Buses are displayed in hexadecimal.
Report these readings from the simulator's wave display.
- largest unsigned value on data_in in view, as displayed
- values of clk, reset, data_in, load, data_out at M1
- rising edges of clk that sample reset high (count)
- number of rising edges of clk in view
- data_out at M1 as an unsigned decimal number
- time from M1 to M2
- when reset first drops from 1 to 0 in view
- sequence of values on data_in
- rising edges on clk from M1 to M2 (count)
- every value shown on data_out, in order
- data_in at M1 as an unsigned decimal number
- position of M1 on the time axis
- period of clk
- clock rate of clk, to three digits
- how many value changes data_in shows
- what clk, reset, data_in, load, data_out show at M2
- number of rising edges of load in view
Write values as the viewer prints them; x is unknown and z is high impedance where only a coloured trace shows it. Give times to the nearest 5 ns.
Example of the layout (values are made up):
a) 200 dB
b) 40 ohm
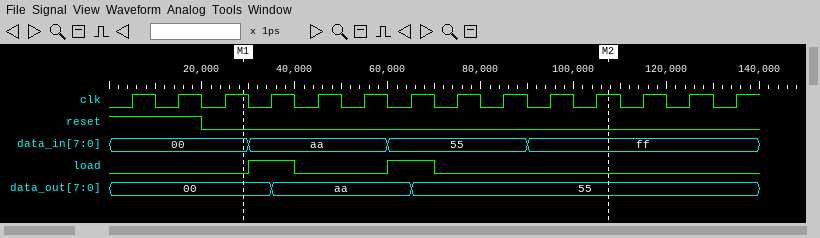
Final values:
a) ff
b) clk=1, reset=0, data_in=00, load=0, data_out=00
c) 2
d) 14
e) 0
f) 80 ns
g) 20 ns
h) 00, aa, 55, ff
i) 8
j) 00, aa, 55
k) 0
l) 30 ns
m) 10 ns
n) 100 MHz
o) 3
p) clk=1, reset=0, data_in=ff, load=0, data_out=55
q) 2
